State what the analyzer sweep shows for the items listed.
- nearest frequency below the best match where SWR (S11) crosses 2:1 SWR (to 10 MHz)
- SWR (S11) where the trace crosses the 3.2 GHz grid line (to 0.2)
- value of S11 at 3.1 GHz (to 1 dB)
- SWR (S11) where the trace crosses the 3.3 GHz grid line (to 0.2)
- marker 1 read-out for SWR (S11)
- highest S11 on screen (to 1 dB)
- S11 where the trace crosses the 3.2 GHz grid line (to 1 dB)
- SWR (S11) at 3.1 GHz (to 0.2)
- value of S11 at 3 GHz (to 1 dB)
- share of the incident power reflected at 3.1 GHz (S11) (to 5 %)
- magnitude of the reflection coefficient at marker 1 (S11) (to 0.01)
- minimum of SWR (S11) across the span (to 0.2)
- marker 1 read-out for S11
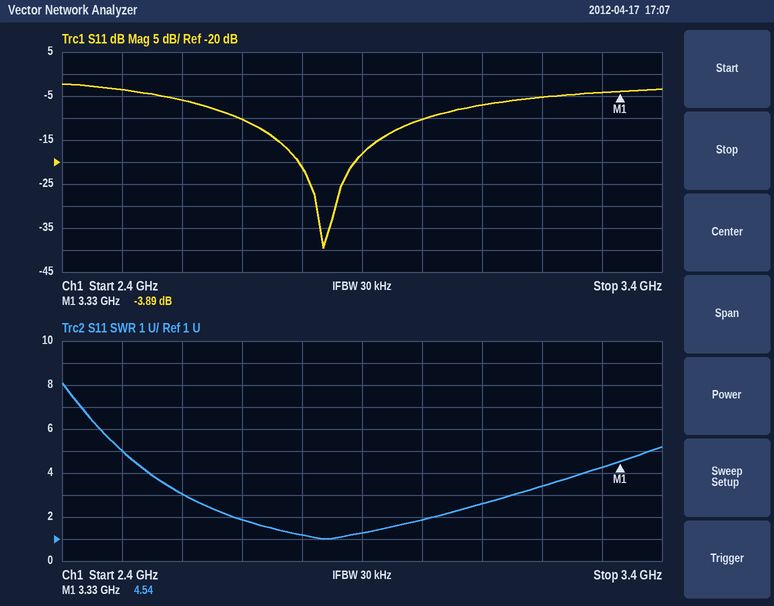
2.69 GHz
3.4
-7 dB
4.2
4.54
-2 dB
-5 dB
2.6
-10 dB
20 %
0.64
1.0
-3.89 dB
